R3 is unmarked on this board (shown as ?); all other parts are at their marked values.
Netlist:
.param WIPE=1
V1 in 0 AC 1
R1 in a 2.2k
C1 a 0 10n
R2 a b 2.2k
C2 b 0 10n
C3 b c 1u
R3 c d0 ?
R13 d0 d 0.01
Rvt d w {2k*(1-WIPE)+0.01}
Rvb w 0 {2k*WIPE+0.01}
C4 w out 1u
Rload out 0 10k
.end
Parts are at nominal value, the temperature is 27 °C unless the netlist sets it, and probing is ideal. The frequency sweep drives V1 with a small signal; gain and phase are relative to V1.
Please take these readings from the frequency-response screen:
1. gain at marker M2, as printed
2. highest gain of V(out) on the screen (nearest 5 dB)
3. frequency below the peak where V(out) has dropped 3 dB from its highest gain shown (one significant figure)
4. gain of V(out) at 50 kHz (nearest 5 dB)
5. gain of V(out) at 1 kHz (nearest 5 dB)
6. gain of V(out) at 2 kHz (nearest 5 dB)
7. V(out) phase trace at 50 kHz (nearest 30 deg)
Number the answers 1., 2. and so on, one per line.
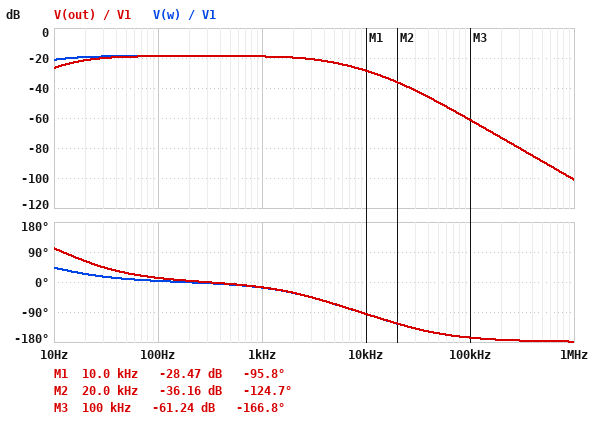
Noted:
1. -36.16 dB
2. -20 dB
3. 20 Hz
4. -50 dB
5. -20 dB
6. -20 dB
7. -150 deg
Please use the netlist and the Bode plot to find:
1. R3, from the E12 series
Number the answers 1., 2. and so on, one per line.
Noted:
1. 8.2 kΩ
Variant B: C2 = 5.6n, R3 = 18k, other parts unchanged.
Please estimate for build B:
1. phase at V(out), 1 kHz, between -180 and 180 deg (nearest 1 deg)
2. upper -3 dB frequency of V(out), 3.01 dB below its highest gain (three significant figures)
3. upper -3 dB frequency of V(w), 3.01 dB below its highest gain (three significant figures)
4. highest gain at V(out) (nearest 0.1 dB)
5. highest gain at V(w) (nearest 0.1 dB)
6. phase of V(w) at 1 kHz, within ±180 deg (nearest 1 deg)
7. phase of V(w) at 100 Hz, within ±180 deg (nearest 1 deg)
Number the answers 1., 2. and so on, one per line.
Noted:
1. -13 deg
2. 4.61 kHz
3. 4.51 kHz
4. -23.2 dB
5. -23.1 dB
6. -14 deg
7. 1 deg
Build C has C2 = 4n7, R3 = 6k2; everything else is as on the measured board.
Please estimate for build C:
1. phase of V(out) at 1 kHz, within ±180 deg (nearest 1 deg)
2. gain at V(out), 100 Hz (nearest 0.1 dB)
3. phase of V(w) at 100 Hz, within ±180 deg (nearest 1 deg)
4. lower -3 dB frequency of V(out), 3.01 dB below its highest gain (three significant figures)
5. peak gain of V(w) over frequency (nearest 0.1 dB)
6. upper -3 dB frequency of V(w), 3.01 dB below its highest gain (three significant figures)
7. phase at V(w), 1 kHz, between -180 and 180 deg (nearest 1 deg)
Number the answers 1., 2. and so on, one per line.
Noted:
1. -10 deg
2. -17.5 dB
3. 5 deg
4. 20.7 Hz
5. -17.4 dB
6. 5.96 kHz
7. -11 deg
